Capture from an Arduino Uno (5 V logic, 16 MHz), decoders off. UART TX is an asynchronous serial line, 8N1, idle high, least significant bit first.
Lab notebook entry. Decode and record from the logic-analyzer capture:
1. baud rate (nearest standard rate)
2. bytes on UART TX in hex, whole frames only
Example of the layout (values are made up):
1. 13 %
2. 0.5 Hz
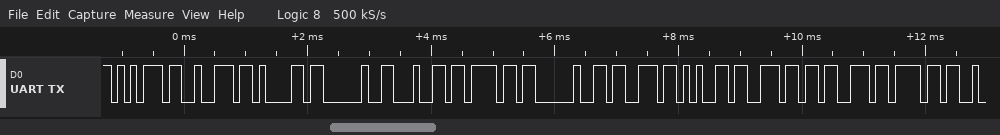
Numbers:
1. 9600 baud
2. 0x75 0x72 0x61 0x20 0x64 0x6F 0x20 0x73 0x65 0x6E 0x73 0x6F
